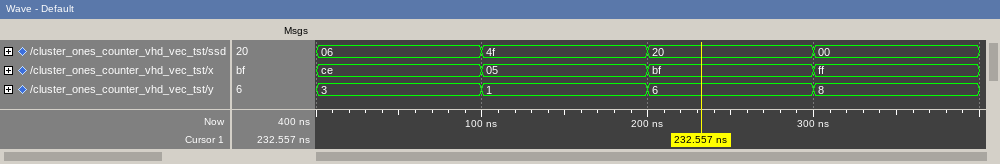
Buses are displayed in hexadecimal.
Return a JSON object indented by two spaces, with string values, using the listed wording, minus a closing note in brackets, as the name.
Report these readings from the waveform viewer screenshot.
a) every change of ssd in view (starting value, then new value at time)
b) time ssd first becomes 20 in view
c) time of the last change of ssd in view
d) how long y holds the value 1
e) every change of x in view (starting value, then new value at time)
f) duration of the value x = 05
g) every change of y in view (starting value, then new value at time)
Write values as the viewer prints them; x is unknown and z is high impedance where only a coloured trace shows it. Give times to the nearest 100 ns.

{
  "every change of ssd in view": "06, 4f at 100 ns, 20 at 200 ns, 00 at 300 ns",
  "time ssd first becomes 20 in view": "200 ns",
  "time of the last change of ssd in view": "300 ns",
  "how long y holds the value 1": "100 ns",
  "every change of x in view": "ce, 05 at 100 ns, bf at 200 ns, ff at 300 ns",
  "duration of the value x = 05": "100 ns",
  "every change of y in view": "3, 1 at 100 ns, 6 at 200 ns, 8 at 300 ns"
}
